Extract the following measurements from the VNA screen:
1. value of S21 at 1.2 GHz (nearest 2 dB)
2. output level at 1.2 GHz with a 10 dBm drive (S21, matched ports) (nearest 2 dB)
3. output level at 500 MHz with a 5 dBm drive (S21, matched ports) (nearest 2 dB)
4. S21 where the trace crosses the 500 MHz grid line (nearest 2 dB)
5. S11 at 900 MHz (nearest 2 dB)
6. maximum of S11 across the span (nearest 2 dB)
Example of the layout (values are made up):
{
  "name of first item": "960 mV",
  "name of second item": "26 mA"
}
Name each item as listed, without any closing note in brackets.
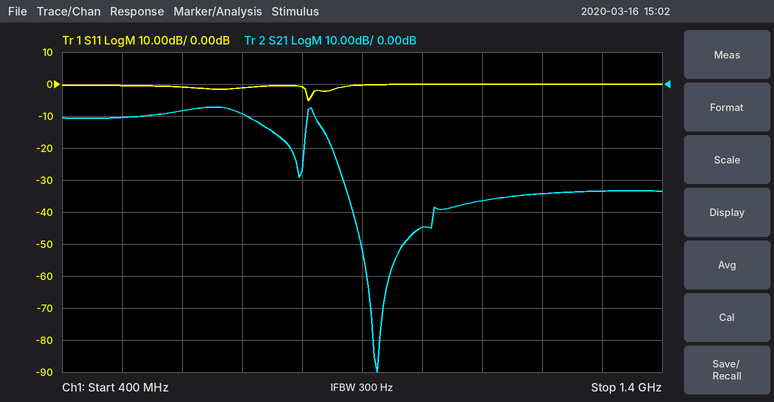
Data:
{
  "value of S21 at 1.2 GHz": "-34 dB",
  "output level at 1.2 GHz with a 10 dBm drive (S21, matched ports)": "-24 dBm",
  "output level at 500 MHz with a 5 dBm drive (S21, matched ports)": "-6 dBm",
  "S21 where the trace crosses the 500 MHz grid line": "-10 dB",
  "S11 at 900 MHz": "0 dB",
  "maximum of S11 across the span": "0 dB"
}
